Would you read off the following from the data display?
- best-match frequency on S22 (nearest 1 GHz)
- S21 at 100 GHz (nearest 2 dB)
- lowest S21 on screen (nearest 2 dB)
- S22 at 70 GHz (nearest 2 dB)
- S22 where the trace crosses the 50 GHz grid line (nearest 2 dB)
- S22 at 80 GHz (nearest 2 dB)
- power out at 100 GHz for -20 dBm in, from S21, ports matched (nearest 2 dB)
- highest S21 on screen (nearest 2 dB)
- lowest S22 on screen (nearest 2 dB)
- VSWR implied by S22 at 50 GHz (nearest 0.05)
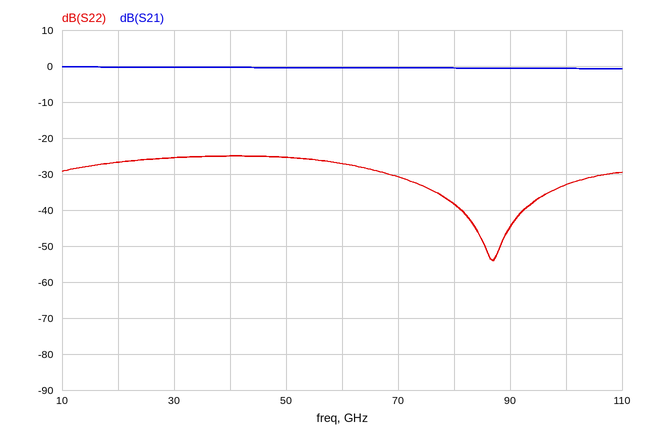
87 GHz
0 dB
0 dB
-30 dB
-26 dB
-38 dB
-20 dBm
0 dB
-54 dB
1.10
